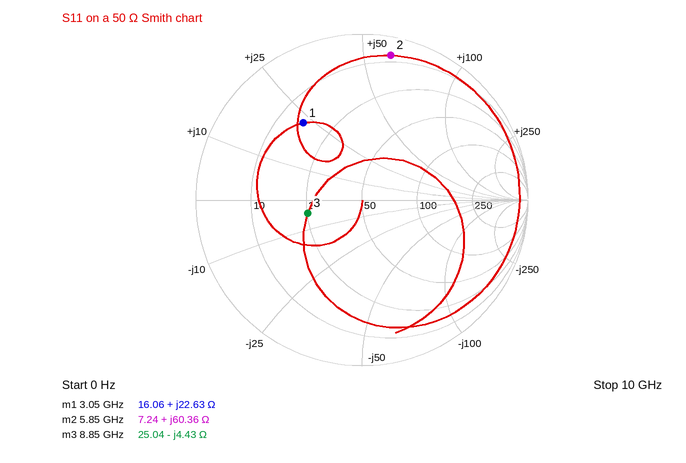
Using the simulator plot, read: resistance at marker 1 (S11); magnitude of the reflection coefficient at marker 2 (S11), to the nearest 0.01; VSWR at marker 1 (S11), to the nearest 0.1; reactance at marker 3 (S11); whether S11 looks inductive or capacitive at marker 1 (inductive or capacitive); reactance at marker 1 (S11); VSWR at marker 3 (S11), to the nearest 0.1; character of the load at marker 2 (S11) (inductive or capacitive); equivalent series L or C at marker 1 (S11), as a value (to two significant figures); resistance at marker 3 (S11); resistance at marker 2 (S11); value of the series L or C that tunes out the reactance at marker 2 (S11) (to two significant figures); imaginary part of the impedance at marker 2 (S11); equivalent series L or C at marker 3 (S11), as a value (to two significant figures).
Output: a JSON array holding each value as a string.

["16.06 Ω", "0.89", "3.8", "-4.43 Ω", "inductive", "+22.63 Ω", "2.0", "inductive", "1.2 nH", "25.04 Ω", "7.24 Ω", "450 fF", "+60.36 Ω", "4.1 pF"]
